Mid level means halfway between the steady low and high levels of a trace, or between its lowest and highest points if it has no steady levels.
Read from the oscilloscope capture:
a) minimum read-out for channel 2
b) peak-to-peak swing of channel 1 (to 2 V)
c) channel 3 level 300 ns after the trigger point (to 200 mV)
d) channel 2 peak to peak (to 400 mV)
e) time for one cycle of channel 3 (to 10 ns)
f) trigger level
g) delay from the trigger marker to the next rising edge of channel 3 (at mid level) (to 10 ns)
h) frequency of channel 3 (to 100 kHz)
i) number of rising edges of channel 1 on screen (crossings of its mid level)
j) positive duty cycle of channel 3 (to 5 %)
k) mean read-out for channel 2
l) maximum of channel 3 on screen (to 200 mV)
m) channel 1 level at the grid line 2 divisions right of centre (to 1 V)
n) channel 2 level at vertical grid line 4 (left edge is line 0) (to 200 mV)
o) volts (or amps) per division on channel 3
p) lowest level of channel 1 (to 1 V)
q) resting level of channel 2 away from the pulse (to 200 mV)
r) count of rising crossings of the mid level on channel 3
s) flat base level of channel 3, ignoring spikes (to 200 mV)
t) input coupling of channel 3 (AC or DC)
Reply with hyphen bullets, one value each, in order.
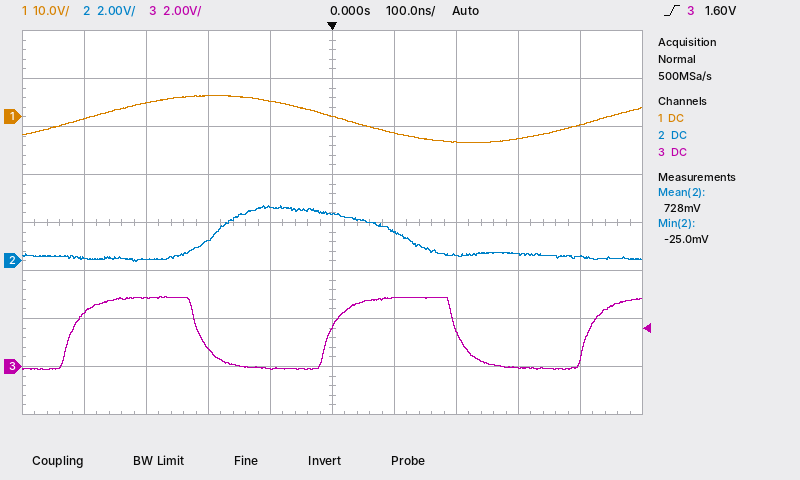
- -25.0 mV
- 10 V
- 0.0 V
- 2.4 V
- 420 ns
- 1.60 V
- 410 ns
- 2.4 MHz
- 2
- 50 %
- 728 mV
- 3.0 V
- -5 V
- 2.2 V
- 2 V
- -5 V
- 200 mV
- 3
- 0.0 V
- DC
